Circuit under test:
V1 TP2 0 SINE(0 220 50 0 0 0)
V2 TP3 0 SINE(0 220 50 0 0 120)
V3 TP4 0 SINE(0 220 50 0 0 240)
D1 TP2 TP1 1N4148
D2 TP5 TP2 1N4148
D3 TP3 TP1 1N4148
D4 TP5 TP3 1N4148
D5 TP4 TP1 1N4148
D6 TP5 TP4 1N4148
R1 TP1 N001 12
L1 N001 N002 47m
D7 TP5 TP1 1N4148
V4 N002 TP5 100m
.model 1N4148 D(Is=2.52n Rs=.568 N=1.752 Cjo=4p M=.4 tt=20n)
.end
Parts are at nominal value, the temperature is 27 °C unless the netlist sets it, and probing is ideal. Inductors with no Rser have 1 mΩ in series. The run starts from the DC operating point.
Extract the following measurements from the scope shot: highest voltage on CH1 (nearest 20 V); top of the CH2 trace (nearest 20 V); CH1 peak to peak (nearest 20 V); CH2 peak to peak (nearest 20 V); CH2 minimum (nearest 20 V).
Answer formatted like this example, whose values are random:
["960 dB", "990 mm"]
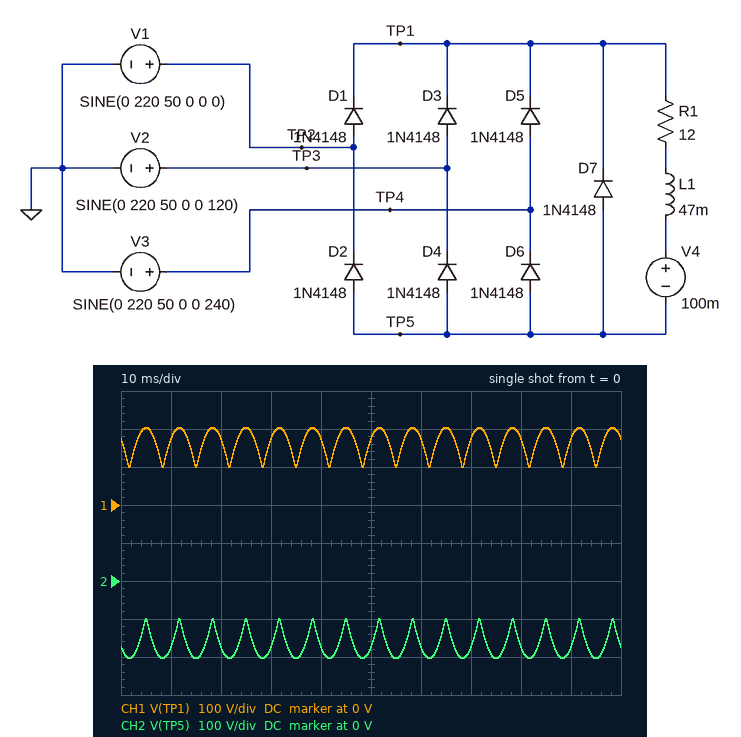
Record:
["200 V", "-100 V", "100 V", "100 V", "-200 V"]
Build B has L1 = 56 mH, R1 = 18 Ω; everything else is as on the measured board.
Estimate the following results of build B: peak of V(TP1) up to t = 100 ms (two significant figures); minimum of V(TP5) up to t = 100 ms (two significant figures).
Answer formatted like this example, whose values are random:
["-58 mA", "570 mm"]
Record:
["210 V", "-210 V"]
